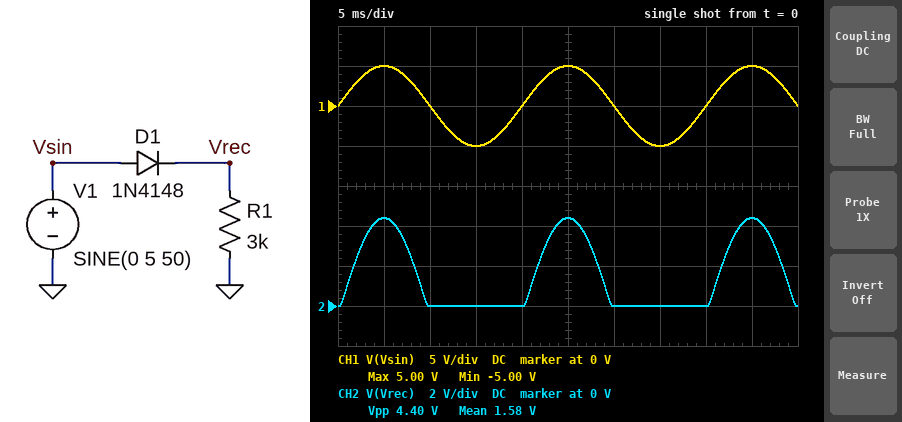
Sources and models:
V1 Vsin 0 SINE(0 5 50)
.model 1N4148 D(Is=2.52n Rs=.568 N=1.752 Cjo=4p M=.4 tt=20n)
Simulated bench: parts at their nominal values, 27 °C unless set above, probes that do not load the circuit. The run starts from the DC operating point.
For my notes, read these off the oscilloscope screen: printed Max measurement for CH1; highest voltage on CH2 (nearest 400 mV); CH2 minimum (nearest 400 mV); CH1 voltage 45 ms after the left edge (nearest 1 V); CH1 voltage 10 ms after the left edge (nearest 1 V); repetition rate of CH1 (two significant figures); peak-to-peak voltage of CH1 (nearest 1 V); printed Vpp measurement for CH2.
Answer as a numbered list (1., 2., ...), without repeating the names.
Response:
1. 5.00 V
2. 4.4 V
3. 0 V
4. 5 V
5. 0 V
6. 50 Hz
7. 10 V
8. 4.40 V
